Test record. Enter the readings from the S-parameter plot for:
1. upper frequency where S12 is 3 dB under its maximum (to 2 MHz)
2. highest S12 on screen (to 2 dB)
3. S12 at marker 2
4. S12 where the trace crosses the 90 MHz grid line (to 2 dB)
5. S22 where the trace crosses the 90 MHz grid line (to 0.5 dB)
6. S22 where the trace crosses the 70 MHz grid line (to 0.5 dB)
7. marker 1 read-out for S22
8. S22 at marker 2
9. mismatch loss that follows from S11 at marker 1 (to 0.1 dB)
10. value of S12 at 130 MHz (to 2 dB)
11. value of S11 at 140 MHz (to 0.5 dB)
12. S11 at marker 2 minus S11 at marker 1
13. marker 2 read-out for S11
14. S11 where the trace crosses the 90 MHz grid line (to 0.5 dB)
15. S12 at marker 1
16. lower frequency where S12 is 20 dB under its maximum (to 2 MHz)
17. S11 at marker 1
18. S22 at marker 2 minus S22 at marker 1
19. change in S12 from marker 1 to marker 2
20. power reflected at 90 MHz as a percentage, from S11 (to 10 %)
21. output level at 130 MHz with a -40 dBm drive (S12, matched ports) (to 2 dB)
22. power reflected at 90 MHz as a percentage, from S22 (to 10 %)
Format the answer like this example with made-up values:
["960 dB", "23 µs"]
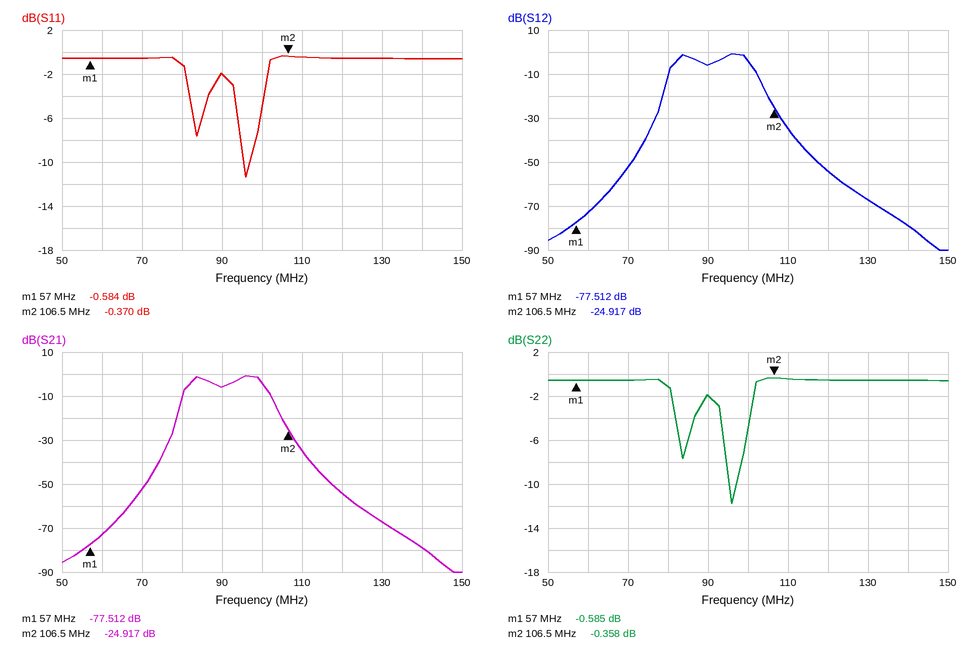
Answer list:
["100 MHz", "0 dB", "-24.917 dB", "-6 dB", "-2.0 dB", "-0.5 dB", "-0.585 dB", "-0.358 dB", "9.0 dB", "-68 dB", "-0.5 dB", "0.214 dB", "-0.370 dB", "-2.0 dB", "-77.512 dB", "78 MHz", "-0.584 dB", "0.227 dB", "52.595 dB", "60 %", "-108 dBm", "60 %"]
